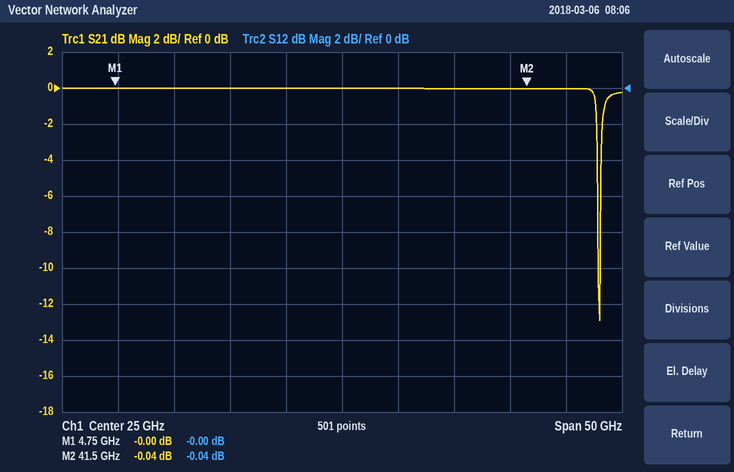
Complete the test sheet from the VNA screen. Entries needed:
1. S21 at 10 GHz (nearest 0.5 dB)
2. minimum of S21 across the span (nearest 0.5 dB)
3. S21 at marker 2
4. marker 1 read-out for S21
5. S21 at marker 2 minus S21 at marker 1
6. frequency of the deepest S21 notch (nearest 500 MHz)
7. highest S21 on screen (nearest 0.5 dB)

0.0 dB
-13.0 dB
-0.04 dB
-0.00 dB
-0.04 dB
48.0 GHz
0.0 dB
